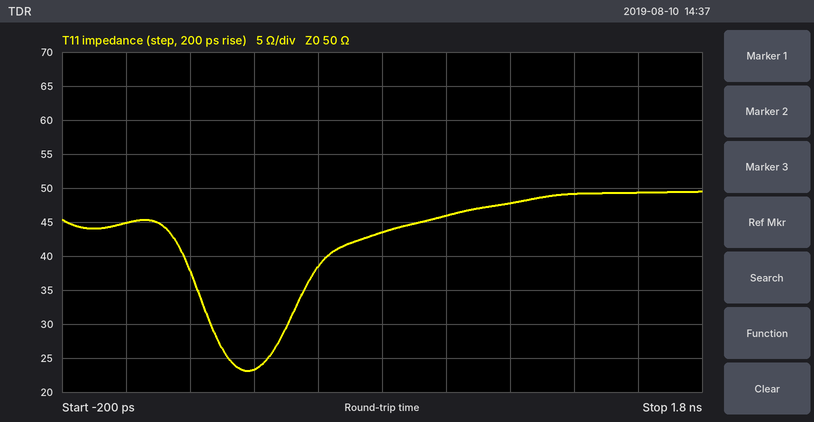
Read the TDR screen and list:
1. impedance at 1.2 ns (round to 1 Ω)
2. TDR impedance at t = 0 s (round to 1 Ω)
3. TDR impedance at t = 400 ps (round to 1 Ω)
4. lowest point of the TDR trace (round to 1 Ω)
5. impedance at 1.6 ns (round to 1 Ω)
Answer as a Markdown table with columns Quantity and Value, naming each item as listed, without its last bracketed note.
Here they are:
| Quantity | Value |
|---|---|
| impedance at 1.2 ns | 48 Ω |
| TDR impedance at t = 0 s | 45 Ω |
| TDR impedance at t = 400 ps | 23 Ω |
| lowest point of the TDR trace | 23 Ω |
| impedance at 1.6 ns | 49 Ω |
